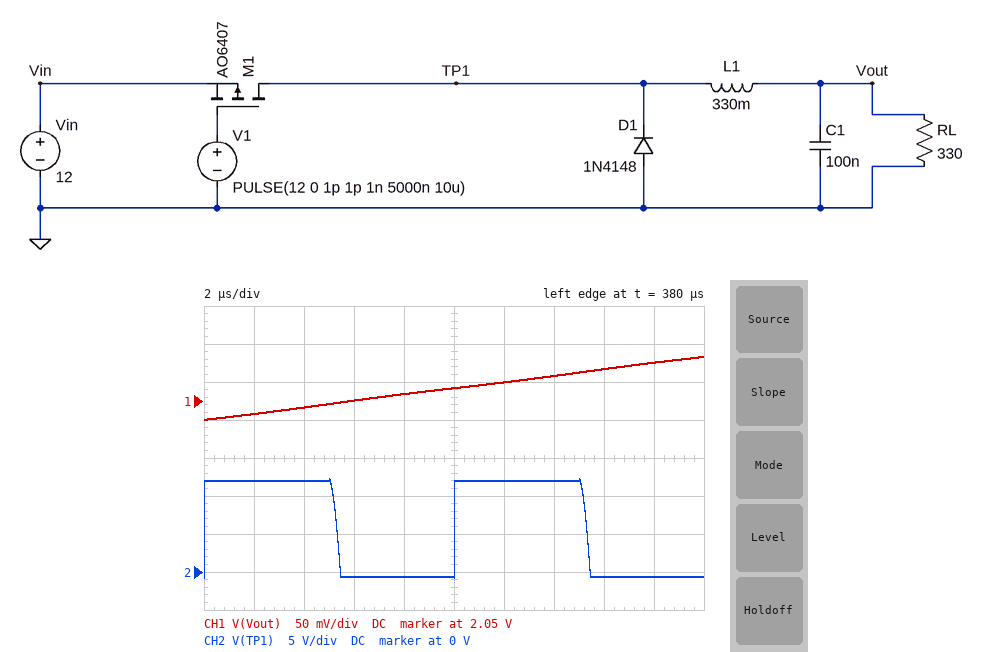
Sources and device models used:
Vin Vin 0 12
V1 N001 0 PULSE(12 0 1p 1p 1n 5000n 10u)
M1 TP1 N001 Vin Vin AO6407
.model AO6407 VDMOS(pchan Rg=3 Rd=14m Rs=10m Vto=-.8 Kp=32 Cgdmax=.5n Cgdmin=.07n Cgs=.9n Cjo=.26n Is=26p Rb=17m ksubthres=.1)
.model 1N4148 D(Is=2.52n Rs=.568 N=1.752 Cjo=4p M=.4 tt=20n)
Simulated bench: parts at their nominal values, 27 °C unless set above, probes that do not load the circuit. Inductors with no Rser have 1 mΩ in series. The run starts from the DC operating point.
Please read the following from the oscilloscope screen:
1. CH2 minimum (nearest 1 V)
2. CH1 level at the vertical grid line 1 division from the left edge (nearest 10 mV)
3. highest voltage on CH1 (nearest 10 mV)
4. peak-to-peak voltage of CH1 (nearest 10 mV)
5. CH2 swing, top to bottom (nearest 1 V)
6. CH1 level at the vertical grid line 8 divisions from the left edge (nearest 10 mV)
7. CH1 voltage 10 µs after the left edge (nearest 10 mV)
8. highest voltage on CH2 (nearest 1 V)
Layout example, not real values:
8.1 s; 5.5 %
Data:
-1 V; 2.03 V; 2.11 V; 80 mV; 13 V; 2.09 V; 2.07 V; 12 V
